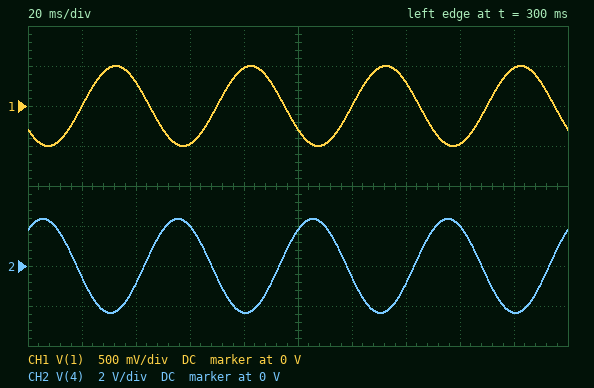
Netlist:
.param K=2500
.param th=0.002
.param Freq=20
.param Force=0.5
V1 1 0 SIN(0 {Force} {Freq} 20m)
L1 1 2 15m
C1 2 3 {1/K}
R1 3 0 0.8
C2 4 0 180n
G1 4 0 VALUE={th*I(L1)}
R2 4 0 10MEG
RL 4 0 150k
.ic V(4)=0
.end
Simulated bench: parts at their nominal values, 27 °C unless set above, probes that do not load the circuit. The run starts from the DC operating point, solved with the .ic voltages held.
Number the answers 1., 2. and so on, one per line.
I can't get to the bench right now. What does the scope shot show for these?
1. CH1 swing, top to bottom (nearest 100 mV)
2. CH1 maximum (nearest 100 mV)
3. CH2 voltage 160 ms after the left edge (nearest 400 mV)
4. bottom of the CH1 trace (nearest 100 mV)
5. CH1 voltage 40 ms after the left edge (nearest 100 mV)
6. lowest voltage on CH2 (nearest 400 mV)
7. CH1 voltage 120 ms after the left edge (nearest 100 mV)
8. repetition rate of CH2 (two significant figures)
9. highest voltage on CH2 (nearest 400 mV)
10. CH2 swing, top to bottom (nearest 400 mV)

1. 1.0 V
2. 500 mV
3. 2.0 V
4. -500 mV
5. 300 mV
6. -2.4 V
7. 0 V
8. 20 Hz
9. 2.4 V
10. 4.8 V
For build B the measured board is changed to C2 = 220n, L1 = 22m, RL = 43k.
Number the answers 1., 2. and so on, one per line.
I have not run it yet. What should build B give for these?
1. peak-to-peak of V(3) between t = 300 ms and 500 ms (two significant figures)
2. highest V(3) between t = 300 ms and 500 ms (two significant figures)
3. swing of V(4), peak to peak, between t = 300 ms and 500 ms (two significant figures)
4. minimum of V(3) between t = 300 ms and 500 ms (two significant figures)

1. 47 mV
2. 23 mV
3. 3.2 V
4. -23 mV
